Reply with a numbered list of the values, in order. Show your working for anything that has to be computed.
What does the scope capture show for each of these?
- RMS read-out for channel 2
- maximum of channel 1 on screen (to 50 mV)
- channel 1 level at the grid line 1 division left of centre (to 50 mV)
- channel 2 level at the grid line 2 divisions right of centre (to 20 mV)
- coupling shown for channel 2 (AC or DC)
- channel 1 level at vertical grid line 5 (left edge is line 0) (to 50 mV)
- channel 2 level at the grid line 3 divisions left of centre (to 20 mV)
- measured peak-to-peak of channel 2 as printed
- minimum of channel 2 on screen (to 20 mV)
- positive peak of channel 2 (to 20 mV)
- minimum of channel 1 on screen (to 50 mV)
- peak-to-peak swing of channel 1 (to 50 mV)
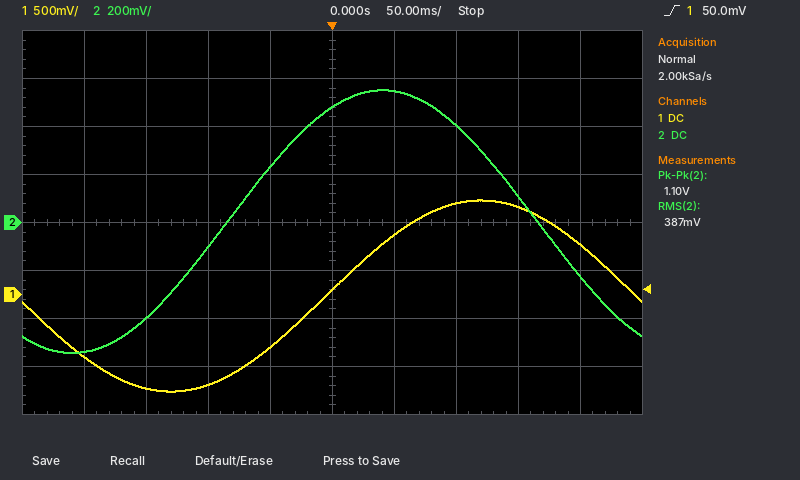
1. 387 mV
2. 1.00 V
3. -550 mV
4. 400 mV
5. DC
6. 50 mV
7. -400 mV
8. 1.10 V
9. -540 mV
10. 560 mV
11. -1.00 V
12. 1.00 V − (-1.00 V) = 2.00 V
